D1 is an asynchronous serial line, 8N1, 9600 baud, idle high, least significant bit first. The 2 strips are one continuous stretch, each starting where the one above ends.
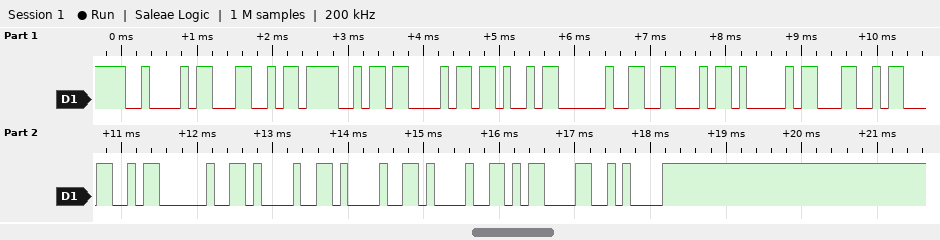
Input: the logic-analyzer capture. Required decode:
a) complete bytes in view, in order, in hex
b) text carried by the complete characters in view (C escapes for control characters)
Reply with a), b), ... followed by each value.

a) 42 4C 4F 43 4B 20 46 41 4C 4C 20 21 21 21 0D 0A
b) "BLOCK FALL !!!\r\n"
